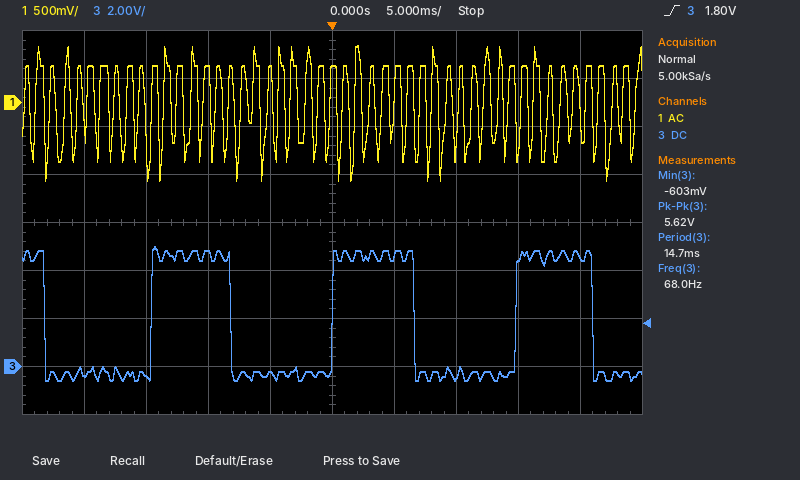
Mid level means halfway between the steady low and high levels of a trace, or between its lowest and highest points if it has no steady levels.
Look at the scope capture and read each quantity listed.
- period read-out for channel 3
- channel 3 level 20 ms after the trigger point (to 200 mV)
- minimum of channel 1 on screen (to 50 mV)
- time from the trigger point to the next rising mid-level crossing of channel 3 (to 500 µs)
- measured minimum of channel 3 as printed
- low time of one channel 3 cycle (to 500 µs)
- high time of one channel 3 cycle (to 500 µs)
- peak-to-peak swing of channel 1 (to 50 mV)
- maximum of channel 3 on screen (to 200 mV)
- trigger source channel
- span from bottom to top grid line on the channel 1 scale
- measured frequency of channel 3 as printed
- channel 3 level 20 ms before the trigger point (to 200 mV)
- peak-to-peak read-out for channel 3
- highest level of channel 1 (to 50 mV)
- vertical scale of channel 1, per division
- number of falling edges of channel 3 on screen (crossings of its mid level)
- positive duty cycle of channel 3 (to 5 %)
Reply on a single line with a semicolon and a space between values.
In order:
14.7 ms; 4.6 V; -800 mV; 15.0 ms; -603 mV; 8.5 ms; 6.5 ms; 1.40 V; 5.0 V; channel 3; 4 V; 68.0 Hz; -200 mV; 5.62 V; 600 mV; 500 mV; 4; 45 %
